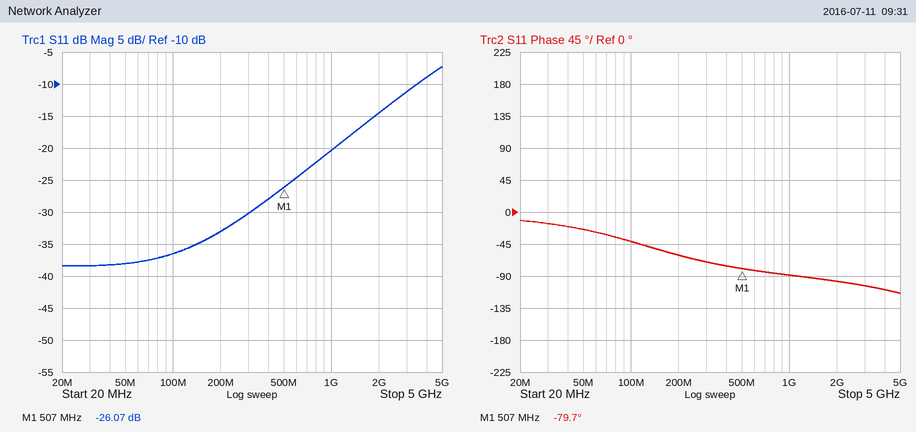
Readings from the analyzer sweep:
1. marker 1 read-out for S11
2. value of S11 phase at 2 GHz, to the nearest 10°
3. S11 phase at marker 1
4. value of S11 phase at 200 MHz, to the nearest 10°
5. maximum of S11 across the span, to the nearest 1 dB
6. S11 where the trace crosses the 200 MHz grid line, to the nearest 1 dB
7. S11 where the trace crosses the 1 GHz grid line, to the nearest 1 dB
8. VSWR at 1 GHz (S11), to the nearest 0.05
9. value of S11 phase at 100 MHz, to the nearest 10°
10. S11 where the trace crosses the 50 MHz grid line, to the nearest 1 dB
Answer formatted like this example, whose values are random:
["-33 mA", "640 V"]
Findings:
["-26.07 dB", "-100°", "-79.7°", "-60°", "-7 dB", "-33 dB", "-20 dB", "1.20", "-40°", "-38 dB"]
